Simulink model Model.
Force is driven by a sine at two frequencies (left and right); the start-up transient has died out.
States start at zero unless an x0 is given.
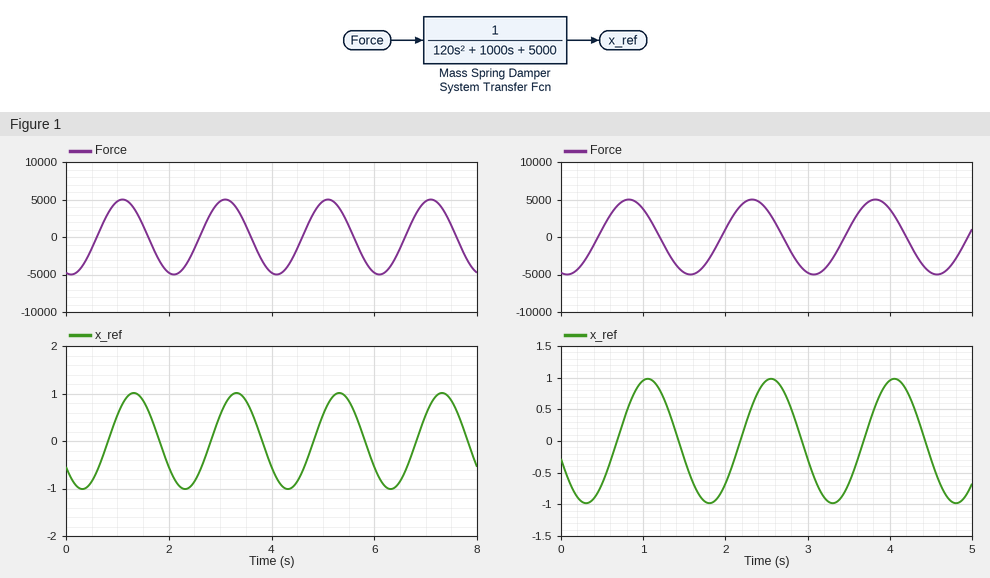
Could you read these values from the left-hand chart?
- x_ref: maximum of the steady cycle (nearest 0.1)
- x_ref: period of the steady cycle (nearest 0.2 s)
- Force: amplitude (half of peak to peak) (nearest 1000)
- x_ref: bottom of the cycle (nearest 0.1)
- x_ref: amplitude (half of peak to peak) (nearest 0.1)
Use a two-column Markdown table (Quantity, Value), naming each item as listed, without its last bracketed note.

| Quantity | Value |
|---|---|
| x_ref: maximum of the steady cycle | 1.0 |
| x_ref: period of the steady cycle | 2.0 s |
| Force: amplitude (half of peak to peak) | 5000 |
| x_ref: bottom of the cycle | -1.0 |
| x_ref: amplitude (half of peak to peak) | 1.0 |
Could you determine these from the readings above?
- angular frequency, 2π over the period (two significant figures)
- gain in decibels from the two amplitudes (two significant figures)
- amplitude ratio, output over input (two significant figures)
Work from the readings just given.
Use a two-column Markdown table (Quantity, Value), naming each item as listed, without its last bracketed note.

| Quantity | Value |
|---|---|
| angular frequency, 2π over the period | 3.1 rad/s |
| gain in decibels from the two amplitudes | -74 dB |
| amplitude ratio, output over input | 0.00020 |
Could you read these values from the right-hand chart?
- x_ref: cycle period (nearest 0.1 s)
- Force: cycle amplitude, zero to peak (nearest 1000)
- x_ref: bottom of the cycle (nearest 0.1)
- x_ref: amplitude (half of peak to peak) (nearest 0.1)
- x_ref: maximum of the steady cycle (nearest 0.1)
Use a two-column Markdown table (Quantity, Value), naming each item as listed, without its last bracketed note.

| Quantity | Value |
|---|---|
| x_ref: cycle period | 1.5 s |
| Force: cycle amplitude, zero to peak | 5000 |
| x_ref: bottom of the cycle | -1.0 |
| x_ref: amplitude (half of peak to peak) | 1.0 |
| x_ref: maximum of the steady cycle | 1.0 |
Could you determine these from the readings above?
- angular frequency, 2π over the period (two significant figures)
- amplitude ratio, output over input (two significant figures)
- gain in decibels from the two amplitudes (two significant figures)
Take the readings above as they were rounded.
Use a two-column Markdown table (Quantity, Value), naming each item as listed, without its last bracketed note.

| Quantity | Value |
|---|---|
| angular frequency, 2π over the period | 4.2 rad/s |
| amplitude ratio, output over input | 0.00020 |
| gain in decibels from the two amplitudes | -74 dB |
